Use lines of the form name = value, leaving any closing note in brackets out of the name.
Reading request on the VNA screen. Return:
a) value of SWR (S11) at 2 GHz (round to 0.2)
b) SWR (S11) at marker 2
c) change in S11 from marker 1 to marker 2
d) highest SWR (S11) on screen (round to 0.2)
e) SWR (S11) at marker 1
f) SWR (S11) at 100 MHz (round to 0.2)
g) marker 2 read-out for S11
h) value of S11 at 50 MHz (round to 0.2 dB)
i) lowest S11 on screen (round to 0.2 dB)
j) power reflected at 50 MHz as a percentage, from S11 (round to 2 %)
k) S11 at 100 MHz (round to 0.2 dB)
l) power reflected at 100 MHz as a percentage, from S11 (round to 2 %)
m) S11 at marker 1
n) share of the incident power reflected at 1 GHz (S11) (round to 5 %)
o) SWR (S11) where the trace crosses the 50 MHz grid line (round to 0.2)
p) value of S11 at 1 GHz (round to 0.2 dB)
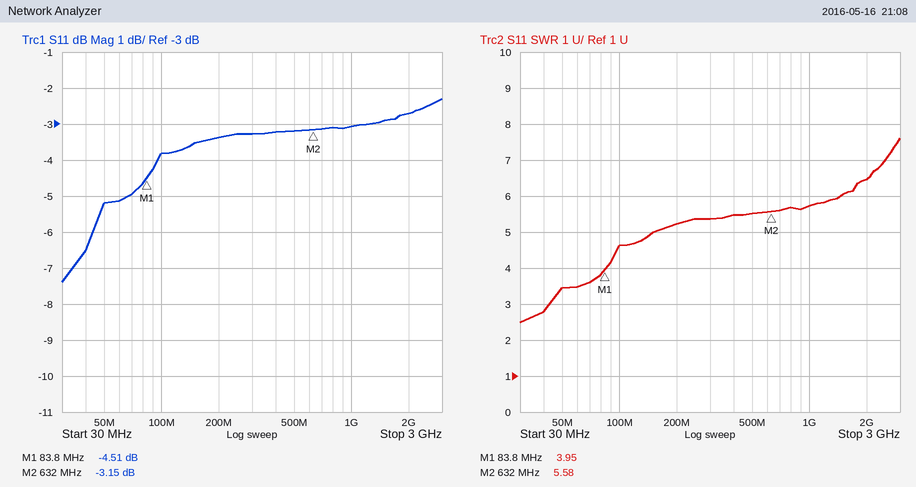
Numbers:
value of SWR (S11) at 2 GHz = 6.4
SWR (S11) at marker 2 = 5.58
change in S11 from marker 1 to marker 2 = 1.36 dB
highest SWR (S11) on screen = 7.6
SWR (S11) at marker 1 = 3.95
SWR (S11) at 100 MHz = 4.6
marker 2 read-out for S11 = -3.15 dB
value of S11 at 50 MHz = -5.2 dB
lowest S11 on screen = -7.4 dB
power reflected at 50 MHz as a percentage, from S11 = 30 %
S11 at 100 MHz = -3.8 dB
power reflected at 100 MHz as a percentage, from S11 = 42 %
S11 at marker 1 = -4.51 dB
share of the incident power reflected at 1 GHz (S11) = 50 %
SWR (S11) where the trace crosses the 50 MHz grid line = 3.4
value of S11 at 1 GHz = -3.0 dB
